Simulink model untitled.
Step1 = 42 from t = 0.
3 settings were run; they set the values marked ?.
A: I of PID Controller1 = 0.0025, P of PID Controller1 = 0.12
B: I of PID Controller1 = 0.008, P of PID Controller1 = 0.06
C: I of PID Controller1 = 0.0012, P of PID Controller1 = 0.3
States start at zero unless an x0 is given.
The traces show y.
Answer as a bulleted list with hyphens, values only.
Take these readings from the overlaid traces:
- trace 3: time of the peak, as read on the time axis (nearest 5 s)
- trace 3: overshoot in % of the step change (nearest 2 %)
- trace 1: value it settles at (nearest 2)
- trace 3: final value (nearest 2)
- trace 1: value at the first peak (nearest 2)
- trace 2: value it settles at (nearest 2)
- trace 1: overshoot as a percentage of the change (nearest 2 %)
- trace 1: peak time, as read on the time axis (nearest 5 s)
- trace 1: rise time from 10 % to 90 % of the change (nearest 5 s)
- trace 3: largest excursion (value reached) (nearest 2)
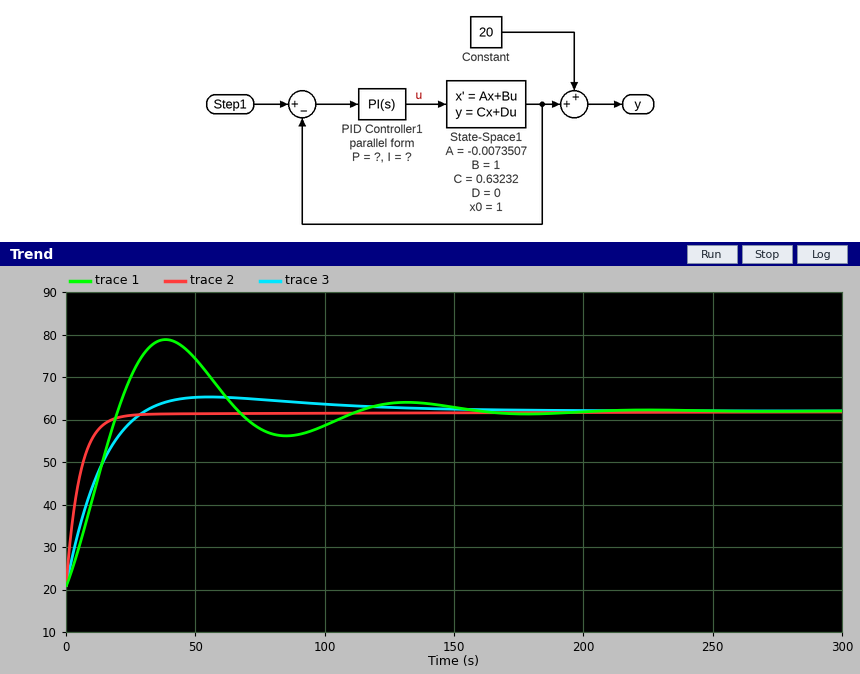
- 55 s
- 8 %
- 62
- 62
- 78
- 62
- 40 %
- 40 s
- 15 s
- 66
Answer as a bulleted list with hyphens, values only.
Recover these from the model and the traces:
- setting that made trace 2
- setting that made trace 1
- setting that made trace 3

- C
- B
- A
